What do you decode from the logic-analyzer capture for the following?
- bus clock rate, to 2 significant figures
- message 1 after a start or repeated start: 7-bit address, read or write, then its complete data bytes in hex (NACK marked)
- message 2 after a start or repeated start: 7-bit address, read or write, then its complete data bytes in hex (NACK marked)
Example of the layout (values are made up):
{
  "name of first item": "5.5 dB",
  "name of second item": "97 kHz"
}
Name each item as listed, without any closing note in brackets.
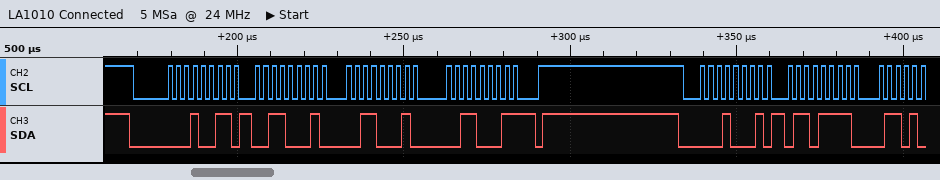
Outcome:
{
  "bus clock rate, to 2 significant figures": "400 kHz",
  "message 1 after a start or repeated start: 7-bit address, read or write, then its complete data bytes in hex": "0x09 read: 31 31 31 NACK",
  "message 2 after a start or repeated start: 7-bit address, read or write, then its complete data bytes in hex": "0x08 read: 6F"
}
